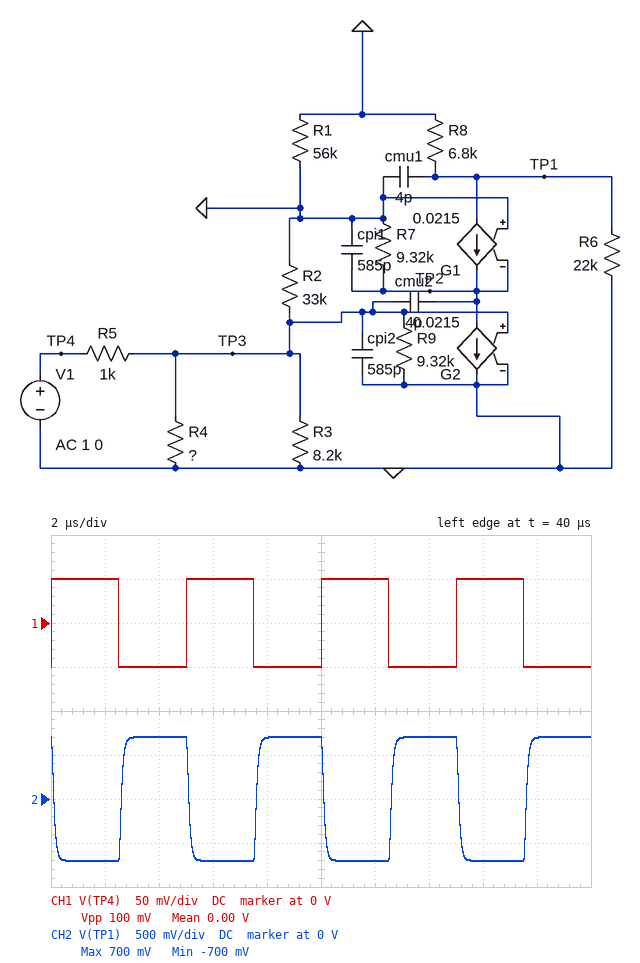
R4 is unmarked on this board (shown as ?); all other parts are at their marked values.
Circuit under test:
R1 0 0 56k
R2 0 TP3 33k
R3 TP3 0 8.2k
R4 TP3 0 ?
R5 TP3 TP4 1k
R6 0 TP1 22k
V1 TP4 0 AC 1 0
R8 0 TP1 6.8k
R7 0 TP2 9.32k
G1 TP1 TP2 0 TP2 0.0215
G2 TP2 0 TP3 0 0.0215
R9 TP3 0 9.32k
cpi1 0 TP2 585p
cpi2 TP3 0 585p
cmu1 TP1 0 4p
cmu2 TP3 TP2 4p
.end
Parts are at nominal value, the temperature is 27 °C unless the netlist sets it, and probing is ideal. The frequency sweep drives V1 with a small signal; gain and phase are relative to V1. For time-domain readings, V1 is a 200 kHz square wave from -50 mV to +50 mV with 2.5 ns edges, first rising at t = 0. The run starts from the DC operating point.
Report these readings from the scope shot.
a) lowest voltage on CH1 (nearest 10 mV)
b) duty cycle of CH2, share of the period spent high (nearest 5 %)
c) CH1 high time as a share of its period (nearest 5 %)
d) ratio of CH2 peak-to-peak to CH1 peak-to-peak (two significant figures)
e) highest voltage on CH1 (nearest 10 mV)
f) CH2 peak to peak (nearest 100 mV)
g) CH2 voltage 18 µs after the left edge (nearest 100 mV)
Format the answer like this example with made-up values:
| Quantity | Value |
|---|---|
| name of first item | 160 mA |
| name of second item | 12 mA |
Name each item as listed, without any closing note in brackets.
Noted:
| Quantity | Value |
|---|---|
| lowest voltage on CH1 | -50 mV |
| duty cycle of CH2, share of the period spent high | 50 % |
| CH1 high time as a share of its period | 50 % |
| ratio of CH2 peak-to-peak to CH1 peak-to-peak | 14 |
| highest voltage on CH1 | 50 mV |
| CH2 peak to peak | 1.4 V |
| CH2 voltage 18 µs after the left edge | 700 mV |
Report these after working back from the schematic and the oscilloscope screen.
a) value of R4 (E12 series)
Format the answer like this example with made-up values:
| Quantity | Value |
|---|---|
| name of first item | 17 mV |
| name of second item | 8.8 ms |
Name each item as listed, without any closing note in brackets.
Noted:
| Quantity | Value |
|---|---|
| value of R4 | 150 Ω |
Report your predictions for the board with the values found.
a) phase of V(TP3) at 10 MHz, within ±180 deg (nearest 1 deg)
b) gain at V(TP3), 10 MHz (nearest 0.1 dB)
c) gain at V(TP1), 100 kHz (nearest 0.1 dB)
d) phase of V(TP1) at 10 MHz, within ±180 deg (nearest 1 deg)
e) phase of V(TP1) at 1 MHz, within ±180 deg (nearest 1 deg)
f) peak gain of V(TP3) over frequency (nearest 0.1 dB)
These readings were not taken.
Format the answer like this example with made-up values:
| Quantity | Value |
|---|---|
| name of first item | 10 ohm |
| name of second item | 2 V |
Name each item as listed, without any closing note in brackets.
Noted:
| Quantity | Value |
|---|---|
| phase of V(TP3) at 10 MHz, within ±180 deg | -78 deg |
| gain at V(TP3), 10 MHz | -31.6 dB |
| gain at V(TP1), 100 kHz | 22.9 dB |
| phase of V(TP1) at 10 MHz, within ±180 deg | -11 deg |
| phase of V(TP1) at 1 MHz, within ±180 deg | 138 deg |
| peak gain of V(TP3) over frequency | -18.0 dB |
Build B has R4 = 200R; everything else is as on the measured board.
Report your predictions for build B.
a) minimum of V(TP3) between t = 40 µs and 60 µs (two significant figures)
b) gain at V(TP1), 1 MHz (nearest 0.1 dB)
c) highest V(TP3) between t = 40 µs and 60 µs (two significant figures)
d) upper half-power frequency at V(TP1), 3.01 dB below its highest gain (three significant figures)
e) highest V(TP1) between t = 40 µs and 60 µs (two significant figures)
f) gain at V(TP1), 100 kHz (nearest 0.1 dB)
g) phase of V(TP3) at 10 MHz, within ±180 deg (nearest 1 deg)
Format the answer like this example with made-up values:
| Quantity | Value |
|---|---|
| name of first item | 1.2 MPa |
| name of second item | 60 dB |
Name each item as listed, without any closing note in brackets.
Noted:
| Quantity | Value |
|---|---|
| minimum of V(TP3) between t = 40 µs and 60 µs | -8.0 mV |
| gain at V(TP1), 1 MHz | 23.5 dB |
| highest V(TP3) between t = 40 µs and 60 µs | 8.0 mV |
| upper half-power frequency at V(TP1), 3.01 dB below its highest gain | 1.51 MHz |
| highest V(TP1) between t = 40 µs and 60 µs | 890 mV |
| gain at V(TP1), 100 kHz | 25.0 dB |
| phase of V(TP3) at 10 MHz, within ±180 deg | -80 deg |
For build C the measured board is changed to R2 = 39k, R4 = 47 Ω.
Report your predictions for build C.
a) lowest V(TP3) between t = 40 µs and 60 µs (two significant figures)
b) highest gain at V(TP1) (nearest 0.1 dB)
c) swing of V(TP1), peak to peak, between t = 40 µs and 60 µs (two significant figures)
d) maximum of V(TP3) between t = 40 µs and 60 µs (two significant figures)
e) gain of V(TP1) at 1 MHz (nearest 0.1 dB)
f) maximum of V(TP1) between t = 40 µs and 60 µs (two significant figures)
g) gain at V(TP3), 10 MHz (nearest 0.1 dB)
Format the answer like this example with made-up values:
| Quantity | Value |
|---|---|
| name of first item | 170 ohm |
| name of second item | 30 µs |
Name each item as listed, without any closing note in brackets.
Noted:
| Quantity | Value |
|---|---|
| lowest V(TP3) between t = 40 µs and 60 µs | -2.2 mV |
| highest gain at V(TP1) | 13.9 dB |
| swing of V(TP1), peak to peak, between t = 40 µs and 60 µs | 490 mV |
| maximum of V(TP3) between t = 40 µs and 60 µs | 2.2 mV |
| gain of V(TP1) at 1 MHz | 13.5 dB |
| maximum of V(TP1) between t = 40 µs and 60 µs | 250 mV |
| gain at V(TP3), 10 MHz | -32.8 dB |
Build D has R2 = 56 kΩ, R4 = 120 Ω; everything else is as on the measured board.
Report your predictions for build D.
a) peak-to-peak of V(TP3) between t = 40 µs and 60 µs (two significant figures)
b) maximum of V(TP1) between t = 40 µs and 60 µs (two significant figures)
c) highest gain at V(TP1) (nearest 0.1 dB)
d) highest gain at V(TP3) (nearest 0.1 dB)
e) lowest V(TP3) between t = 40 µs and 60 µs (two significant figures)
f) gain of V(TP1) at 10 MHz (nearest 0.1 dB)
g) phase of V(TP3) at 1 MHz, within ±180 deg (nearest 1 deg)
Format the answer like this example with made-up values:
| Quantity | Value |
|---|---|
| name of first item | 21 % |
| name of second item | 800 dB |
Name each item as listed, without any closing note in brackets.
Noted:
| Quantity | Value |
|---|---|
| peak-to-peak of V(TP3) between t = 40 µs and 60 µs | 10 mV |
| maximum of V(TP1) between t = 40 µs and 60 µs | 580 mV |
| highest gain at V(TP1) | 21.3 dB |
| highest gain at V(TP3) | -19.6 dB |
| lowest V(TP3) between t = 40 µs and 60 µs | -5.2 mV |
| gain of V(TP1) at 10 MHz | -1.0 dB |
| phase of V(TP3) at 1 MHz, within ±180 deg | -21 deg |
